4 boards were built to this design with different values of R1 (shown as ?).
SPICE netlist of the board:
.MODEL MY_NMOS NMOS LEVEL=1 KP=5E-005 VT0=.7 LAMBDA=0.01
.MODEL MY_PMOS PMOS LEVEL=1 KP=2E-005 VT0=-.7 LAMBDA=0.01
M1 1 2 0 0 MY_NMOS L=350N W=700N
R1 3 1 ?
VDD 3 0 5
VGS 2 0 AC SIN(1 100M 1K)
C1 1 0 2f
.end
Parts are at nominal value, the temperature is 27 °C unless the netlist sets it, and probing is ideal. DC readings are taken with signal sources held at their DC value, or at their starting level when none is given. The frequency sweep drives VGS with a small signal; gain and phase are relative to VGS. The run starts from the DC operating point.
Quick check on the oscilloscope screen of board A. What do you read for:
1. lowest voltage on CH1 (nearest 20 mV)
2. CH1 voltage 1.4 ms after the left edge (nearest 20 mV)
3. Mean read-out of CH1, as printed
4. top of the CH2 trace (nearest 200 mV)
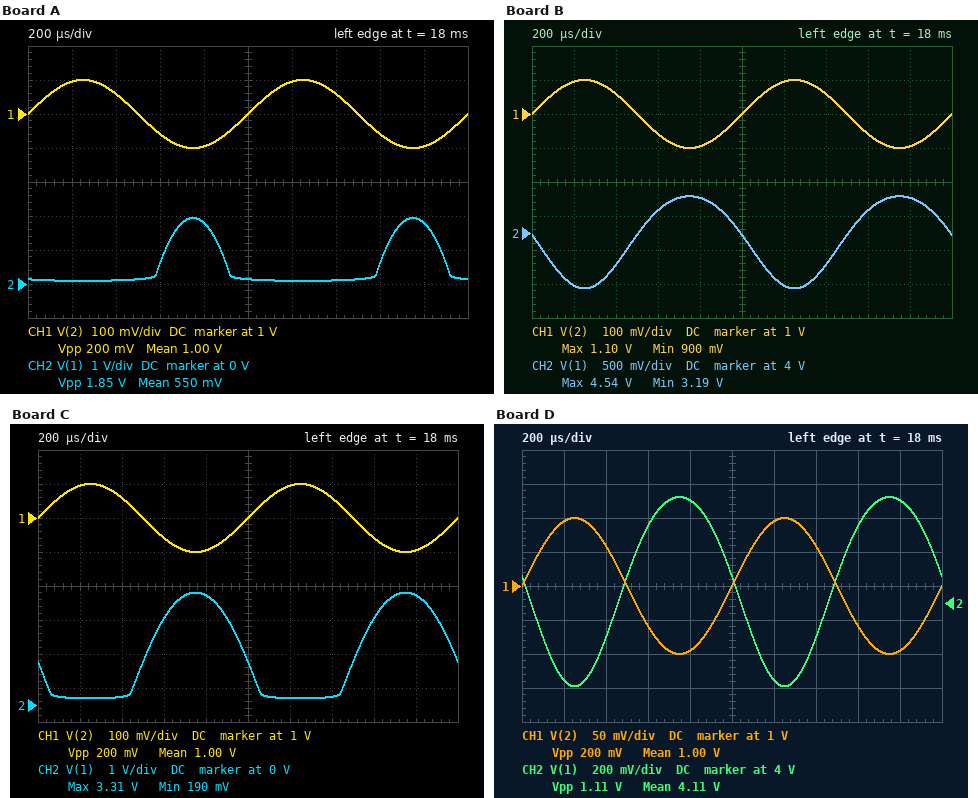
900 mV
1.06 V
1.00 V
2.0 V
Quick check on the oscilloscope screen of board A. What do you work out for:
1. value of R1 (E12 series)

1.5 MΩ
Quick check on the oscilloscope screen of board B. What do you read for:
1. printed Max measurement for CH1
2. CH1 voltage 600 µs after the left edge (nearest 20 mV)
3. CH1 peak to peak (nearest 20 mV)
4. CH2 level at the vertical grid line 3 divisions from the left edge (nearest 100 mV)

1.10 V
940 mV
200 mV
4.3 V
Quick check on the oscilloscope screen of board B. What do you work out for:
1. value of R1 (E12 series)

220 kΩ
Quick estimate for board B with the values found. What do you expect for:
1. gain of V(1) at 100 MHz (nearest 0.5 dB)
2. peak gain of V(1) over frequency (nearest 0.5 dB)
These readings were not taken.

16.5 dB
16.5 dB
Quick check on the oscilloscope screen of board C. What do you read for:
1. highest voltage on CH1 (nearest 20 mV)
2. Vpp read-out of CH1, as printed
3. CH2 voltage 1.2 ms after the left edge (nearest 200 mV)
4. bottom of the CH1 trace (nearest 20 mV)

1.10 V
200 mV
200 mV
900 mV
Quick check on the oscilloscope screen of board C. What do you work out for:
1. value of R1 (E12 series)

820 kΩ
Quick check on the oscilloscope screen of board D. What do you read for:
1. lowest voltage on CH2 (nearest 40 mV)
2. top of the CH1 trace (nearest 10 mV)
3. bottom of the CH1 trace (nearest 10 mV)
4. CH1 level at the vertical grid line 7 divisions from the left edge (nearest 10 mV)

3.52 V
1.10 V
900 mV
1.06 V
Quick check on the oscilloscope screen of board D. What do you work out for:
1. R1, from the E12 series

180 kΩ
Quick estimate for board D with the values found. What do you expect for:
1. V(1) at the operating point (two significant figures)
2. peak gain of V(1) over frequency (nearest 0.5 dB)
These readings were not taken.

4.2 V
15.0 dB
